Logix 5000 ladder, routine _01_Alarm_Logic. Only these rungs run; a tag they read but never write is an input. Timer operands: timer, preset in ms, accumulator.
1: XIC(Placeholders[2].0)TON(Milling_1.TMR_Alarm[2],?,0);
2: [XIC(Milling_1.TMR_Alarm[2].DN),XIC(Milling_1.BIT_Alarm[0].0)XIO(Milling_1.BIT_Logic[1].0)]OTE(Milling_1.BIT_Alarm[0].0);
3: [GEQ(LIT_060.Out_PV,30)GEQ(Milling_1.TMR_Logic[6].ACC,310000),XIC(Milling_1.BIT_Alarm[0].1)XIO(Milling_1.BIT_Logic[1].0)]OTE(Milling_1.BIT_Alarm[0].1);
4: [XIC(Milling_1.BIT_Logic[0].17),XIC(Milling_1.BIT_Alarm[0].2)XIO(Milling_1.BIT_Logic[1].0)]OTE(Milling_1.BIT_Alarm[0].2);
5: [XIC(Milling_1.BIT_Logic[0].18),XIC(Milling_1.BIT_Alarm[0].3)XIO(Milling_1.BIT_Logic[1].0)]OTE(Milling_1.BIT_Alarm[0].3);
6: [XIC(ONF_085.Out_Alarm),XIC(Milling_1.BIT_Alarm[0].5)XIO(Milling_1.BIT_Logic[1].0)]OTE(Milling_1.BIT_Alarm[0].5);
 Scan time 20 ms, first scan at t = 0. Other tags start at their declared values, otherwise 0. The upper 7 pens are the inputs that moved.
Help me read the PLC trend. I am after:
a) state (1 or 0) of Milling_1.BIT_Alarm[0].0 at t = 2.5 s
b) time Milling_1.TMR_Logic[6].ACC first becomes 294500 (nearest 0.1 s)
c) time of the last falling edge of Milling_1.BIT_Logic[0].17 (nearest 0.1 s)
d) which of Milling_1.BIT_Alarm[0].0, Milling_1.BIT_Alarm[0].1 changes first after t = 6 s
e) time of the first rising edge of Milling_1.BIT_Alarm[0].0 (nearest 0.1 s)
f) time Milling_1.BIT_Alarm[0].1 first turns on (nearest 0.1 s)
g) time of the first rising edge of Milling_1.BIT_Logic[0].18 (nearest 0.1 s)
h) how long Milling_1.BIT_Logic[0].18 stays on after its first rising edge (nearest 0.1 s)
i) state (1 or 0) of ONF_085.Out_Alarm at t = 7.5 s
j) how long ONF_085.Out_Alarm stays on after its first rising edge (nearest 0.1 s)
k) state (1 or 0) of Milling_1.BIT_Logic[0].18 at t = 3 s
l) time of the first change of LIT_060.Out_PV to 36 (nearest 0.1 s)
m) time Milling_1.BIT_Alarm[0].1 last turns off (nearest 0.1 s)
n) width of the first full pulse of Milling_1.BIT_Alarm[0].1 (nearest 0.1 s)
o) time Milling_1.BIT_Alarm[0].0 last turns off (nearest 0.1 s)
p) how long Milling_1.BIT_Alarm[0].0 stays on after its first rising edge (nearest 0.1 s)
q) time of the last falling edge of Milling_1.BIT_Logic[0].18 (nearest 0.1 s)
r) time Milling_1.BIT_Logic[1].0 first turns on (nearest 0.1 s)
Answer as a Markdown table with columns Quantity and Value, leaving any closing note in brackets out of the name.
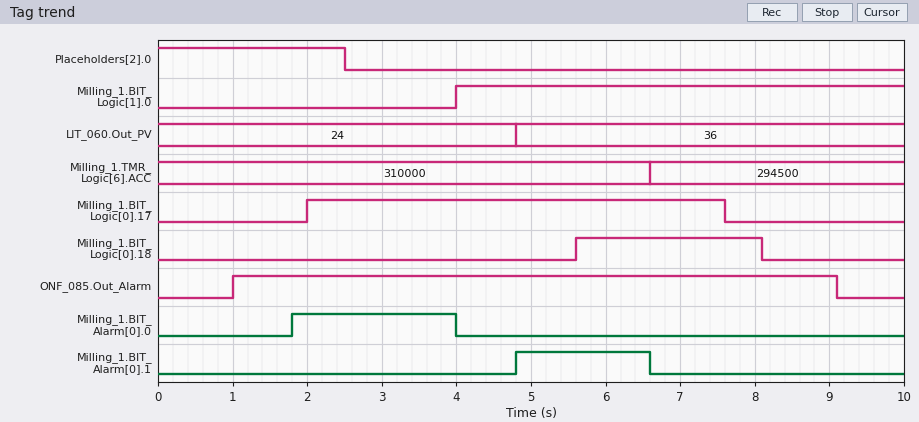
| Quantity | Value |
|---|---|
| state (1 or 0) of Milling_1.BIT_Alarm[0].0 at t = 2.5 s | 1 |
| time Milling_1.TMR_Logic[6].ACC first becomes 294500 | 6.6 s |
| time of the last falling edge of Milling_1.BIT_Logic[0].17 | 7.6 s |
| which of Milling_1.BIT_Alarm[0].0, Milling_1.BIT_Alarm[0].1 changes first after t = 6 s | Milling_1.BIT_Alarm[0].1 |
| time of the first rising edge of Milling_1.BIT_Alarm[0].0 | 1.8 s |
| time Milling_1.BIT_Alarm[0].1 first turns on | 4.8 s |
| time of the first rising edge of Milling_1.BIT_Logic[0].18 | 5.6 s |
| how long Milling_1.BIT_Logic[0].18 stays on after its first rising edge | 2.5 s |
| state (1 or 0) of ONF_085.Out_Alarm at t = 7.5 s | 1 |
| how long ONF_085.Out_Alarm stays on after its first rising edge | 8.1 s |
| state (1 or 0) of Milling_1.BIT_Logic[0].18 at t = 3 s | 0 |
| time of the first change of LIT_060.Out_PV to 36 | 4.8 s |
| time Milling_1.BIT_Alarm[0].1 last turns off | 6.6 s |
| width of the first full pulse of Milling_1.BIT_Alarm[0].1 | 1.8 s |
| time Milling_1.BIT_Alarm[0].0 last turns off | 4.0 s |
| how long Milling_1.BIT_Alarm[0].0 stays on after its first rising edge | 2.2 s |
| time of the last falling edge of Milling_1.BIT_Logic[0].18 | 8.1 s |
| time Milling_1.BIT_Logic[1].0 first turns on | 4.0 s |
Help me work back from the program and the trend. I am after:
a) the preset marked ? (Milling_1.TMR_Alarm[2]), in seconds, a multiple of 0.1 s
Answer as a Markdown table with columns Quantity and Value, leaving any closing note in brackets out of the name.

| Quantity | Value |
|---|---|
| the preset marked ? (Milling_1.TMR_Alarm[2]), in seconds, a multiple of 0.1 s | 1.8 s |
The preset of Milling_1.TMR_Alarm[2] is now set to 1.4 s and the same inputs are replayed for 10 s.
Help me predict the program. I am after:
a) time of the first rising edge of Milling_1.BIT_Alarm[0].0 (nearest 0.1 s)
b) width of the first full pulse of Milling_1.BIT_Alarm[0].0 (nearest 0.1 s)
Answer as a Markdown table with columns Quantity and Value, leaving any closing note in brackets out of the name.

| Quantity | Value |
|---|---|
| time of the first rising edge of Milling_1.BIT_Alarm[0].0 | 1.4 s |
| width of the first full pulse of Milling_1.BIT_Alarm[0].0 | 2.6 s |
